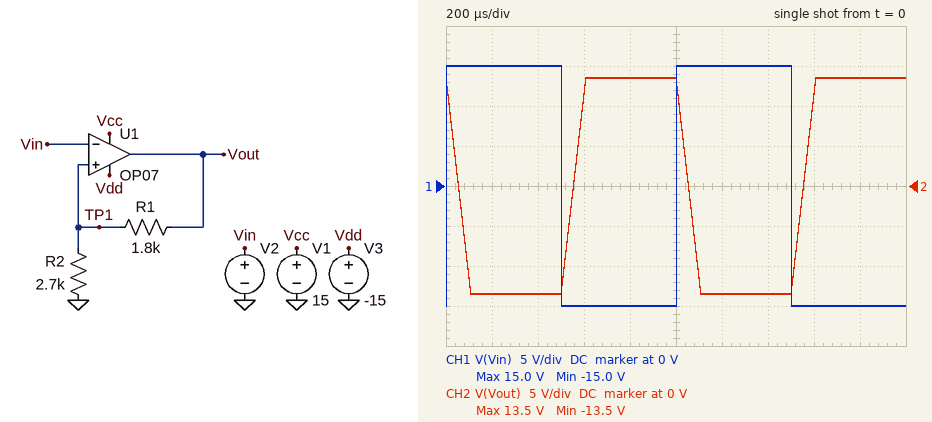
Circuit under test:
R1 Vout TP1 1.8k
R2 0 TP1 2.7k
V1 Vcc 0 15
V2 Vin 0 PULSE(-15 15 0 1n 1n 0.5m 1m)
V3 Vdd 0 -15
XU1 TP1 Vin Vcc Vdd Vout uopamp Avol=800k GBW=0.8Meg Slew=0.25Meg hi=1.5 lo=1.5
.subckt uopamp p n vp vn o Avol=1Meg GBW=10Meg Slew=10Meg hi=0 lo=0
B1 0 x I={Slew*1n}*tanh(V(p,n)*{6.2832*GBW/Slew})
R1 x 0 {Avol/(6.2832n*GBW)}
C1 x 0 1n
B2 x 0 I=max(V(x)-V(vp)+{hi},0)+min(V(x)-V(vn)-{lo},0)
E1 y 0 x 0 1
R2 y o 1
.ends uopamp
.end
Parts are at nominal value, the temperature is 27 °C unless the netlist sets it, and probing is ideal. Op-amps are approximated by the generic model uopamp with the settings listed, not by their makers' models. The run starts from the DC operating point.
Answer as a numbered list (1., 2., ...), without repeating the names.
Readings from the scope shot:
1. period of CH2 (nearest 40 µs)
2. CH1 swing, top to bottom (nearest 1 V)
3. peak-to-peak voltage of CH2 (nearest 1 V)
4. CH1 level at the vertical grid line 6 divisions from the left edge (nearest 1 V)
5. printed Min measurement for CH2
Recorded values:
1. 1.00 ms
2. 30 V
3. 27 V
4. 15 V
5. -13.5 V
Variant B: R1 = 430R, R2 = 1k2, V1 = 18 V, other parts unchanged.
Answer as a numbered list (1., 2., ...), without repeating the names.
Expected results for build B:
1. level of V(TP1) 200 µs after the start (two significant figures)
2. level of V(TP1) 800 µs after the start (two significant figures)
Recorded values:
1. -9.9 V
2. 12 V
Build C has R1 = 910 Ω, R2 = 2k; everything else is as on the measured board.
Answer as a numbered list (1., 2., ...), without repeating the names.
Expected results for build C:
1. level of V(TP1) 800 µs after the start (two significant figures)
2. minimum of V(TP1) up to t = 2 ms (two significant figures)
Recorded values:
1. 9.3 V
2. -9.3 V
